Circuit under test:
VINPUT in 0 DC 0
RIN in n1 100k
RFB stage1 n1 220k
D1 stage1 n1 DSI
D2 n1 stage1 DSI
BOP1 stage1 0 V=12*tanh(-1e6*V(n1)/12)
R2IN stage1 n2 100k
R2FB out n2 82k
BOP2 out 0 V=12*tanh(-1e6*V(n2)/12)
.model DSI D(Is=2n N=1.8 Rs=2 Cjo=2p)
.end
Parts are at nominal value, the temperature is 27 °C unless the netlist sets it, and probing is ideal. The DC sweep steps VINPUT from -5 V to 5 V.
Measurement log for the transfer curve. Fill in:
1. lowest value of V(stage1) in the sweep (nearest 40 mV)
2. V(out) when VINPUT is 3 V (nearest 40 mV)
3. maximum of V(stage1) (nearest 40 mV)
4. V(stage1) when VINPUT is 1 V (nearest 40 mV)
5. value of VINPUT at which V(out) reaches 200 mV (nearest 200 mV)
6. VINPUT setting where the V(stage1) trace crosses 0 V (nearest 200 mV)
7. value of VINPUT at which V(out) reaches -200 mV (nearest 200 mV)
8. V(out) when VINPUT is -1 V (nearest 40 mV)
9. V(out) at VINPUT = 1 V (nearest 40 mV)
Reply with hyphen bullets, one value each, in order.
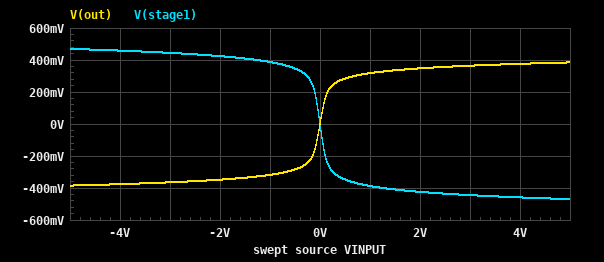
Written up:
- -480 mV
- 360 mV
- 480 mV
- -400 mV
- 200 mV
- 0 V
- -200 mV
- -320 mV
- 320 mV
